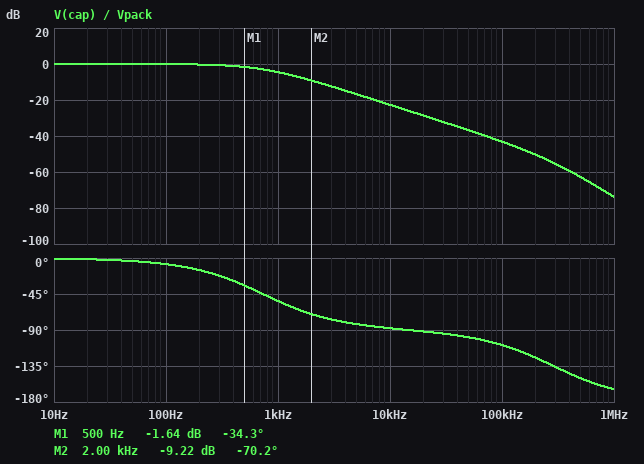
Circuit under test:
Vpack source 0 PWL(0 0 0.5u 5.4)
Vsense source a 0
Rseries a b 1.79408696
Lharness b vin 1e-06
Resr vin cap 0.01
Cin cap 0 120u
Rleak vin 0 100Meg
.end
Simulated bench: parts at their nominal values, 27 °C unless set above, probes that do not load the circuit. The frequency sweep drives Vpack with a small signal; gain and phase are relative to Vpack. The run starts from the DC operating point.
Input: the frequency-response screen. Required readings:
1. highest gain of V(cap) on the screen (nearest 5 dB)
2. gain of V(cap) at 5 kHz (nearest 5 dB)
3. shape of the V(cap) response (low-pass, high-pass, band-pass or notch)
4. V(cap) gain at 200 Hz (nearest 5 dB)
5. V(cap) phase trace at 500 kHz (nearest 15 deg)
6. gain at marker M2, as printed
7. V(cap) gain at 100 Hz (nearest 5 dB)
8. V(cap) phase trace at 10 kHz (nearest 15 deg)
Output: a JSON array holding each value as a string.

["0 dB", "-15 dB", "low-pass", "0 dB", "-150 deg", "-9.22 dB", "0 dB", "-90 deg"]
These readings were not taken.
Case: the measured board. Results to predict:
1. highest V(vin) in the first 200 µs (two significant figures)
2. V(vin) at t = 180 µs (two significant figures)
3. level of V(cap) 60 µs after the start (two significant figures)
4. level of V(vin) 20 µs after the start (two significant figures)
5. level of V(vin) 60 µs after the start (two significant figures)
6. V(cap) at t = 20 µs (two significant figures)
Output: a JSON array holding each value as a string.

["3.3 V", "3.1 V", "1.3 V", "490 mV", "1.3 V", "460 mV"]
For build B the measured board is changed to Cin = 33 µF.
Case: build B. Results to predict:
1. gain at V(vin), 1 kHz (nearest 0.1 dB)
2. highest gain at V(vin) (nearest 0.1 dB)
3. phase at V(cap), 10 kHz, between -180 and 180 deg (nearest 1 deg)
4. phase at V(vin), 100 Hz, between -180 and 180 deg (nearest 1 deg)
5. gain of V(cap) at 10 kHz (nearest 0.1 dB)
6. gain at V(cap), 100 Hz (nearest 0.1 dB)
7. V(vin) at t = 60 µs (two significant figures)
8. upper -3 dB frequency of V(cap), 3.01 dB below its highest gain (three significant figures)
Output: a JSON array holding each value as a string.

["-0.6 dB", "0 dB", "-77 deg", "-2 deg", "-11.7 dB", "0 dB", "3.4 V", "2.70 kHz"]
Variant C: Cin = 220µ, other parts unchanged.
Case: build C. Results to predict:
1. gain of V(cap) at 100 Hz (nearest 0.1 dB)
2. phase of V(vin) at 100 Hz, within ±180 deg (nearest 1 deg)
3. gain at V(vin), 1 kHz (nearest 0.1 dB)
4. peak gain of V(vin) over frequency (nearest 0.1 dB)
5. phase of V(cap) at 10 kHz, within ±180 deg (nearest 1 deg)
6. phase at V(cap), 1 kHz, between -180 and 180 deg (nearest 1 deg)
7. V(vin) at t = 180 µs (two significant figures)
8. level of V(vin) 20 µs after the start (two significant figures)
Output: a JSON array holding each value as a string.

["-0.3 dB", "-14 deg", "-8.6 dB", "0 dB", "-90 deg", "-68 deg", "2.0 V", "280 mV"]
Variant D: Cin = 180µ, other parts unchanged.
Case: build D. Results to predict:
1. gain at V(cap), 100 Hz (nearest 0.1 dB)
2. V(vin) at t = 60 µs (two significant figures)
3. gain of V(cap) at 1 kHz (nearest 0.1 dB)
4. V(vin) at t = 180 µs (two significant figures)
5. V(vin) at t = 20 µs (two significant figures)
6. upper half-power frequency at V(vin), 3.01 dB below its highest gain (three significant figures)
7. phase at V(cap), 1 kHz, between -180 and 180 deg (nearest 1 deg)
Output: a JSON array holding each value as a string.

["-0.2 dB", "930 mV", "-7.1 dB", "2.3 V", "340 mV", "491 Hz", "-64 deg"]
